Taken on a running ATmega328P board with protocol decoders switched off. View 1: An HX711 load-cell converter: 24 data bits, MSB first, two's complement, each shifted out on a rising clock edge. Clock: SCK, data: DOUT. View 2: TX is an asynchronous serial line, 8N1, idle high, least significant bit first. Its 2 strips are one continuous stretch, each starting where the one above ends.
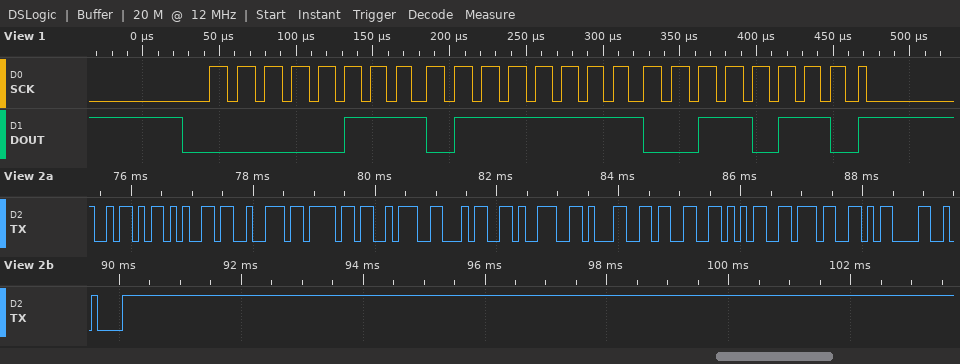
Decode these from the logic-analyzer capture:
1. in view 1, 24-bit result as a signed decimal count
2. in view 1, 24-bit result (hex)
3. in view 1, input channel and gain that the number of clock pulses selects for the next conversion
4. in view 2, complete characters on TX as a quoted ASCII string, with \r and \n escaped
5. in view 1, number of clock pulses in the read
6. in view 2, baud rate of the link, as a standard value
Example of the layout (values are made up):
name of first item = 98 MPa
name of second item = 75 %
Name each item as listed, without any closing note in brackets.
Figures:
in view 1, 24-bit result as a signed decimal count = 491318
in view 1, 24-bit result = 0x077F36
in view 1, input channel and gain that the number of clock pulses selects for the next conversion = channel A, gain 128
in view 2, complete characters on TX as a quoted ASCII string, with \r and \n escaped = "Zero:491357\r\n"
in view 1, number of clock pulses in the read = 25
in view 2, baud rate of the link, as a standard value = 9600 baud
